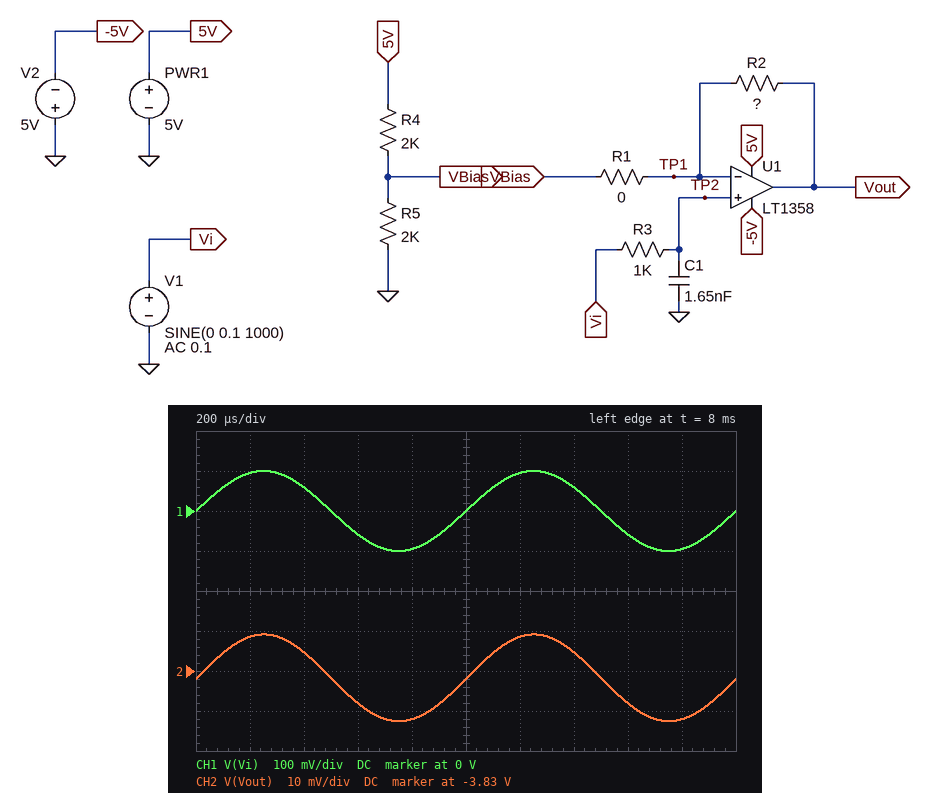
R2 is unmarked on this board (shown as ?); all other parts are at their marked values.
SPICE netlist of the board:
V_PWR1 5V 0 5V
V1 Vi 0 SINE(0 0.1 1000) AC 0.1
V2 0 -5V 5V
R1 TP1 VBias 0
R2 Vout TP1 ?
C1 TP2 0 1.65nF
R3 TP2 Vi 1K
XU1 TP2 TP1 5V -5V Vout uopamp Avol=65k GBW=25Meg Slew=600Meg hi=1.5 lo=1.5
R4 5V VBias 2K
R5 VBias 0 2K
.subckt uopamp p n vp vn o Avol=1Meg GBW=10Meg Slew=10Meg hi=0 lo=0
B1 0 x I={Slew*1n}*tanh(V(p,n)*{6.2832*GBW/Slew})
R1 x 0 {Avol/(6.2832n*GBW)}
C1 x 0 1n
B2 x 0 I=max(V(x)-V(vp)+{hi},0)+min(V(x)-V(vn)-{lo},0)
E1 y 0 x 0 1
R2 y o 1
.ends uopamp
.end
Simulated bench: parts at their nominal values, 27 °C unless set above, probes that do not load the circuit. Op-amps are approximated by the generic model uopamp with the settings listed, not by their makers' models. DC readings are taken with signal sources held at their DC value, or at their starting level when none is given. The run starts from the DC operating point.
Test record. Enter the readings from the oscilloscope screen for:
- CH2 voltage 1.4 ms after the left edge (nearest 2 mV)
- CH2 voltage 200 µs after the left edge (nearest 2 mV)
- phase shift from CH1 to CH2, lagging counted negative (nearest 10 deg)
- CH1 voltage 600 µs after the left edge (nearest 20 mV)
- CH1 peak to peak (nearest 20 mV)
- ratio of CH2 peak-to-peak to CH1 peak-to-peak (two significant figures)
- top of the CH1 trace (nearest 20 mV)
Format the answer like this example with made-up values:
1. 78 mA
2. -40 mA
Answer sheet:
1. -3.826 V
2. -3.822 V
3. 0 deg
4. -60 mV
5. 200 mV
6. 0.11
7. 100 mV
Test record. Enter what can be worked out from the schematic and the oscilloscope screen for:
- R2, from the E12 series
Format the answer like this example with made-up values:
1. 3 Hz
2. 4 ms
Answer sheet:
1. 22 kΩ
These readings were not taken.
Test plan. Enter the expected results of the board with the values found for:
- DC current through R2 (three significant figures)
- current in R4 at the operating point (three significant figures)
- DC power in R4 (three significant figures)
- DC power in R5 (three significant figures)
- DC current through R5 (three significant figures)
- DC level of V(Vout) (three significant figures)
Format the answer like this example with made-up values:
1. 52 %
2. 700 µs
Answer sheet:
1. 282 µA
2. 1.31 mA
3. 3.43 mW
4. 2.84 mW
5. 1.19 mA
6. -3.83 V
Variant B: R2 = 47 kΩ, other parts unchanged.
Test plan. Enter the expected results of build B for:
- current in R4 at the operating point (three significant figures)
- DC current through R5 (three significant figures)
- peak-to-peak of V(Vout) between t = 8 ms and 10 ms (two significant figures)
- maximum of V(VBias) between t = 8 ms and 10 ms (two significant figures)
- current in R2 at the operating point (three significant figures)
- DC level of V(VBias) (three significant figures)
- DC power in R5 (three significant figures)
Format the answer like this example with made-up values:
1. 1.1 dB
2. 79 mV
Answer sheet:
1. 1.26 mA
2. 1.24 mA
3. 21 mV
4. 2.5 V
5. 134 µA
6. 2.48 V
7. 3.07 mW
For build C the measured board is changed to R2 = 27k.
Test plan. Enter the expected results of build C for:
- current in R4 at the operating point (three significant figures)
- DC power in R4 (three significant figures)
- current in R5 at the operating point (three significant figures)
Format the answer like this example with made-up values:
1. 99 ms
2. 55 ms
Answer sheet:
1. 1.29 mA
2. 3.34 mW
3. 1.21 mA
